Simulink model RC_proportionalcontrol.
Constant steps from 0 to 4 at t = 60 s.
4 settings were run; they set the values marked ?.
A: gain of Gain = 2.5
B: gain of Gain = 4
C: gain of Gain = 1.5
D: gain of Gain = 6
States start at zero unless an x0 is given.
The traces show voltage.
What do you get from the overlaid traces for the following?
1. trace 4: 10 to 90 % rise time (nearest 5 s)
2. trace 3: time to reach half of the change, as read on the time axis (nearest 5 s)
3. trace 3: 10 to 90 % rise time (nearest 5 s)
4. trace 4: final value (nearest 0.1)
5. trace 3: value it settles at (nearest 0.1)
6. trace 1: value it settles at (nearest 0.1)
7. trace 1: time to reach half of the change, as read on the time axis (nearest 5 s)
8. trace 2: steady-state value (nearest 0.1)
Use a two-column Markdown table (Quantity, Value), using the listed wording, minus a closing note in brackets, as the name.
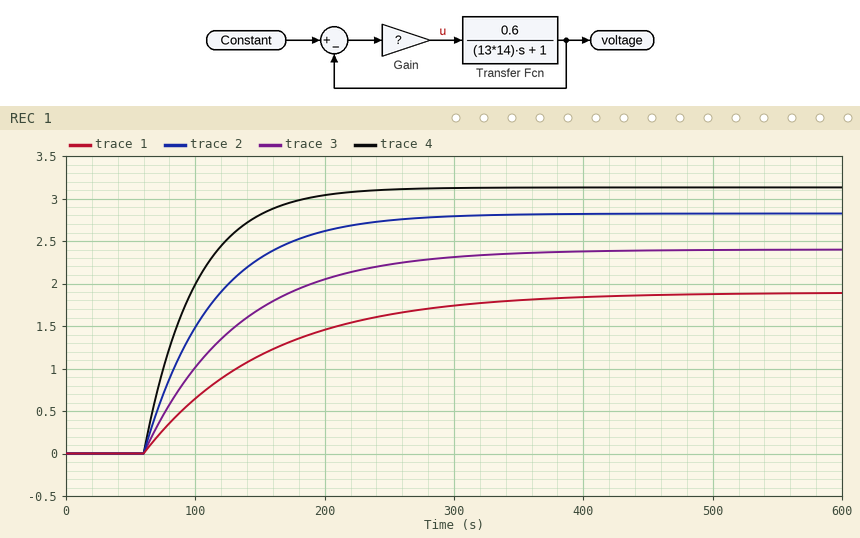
| Quantity | Value |
|---|---|
| trace 4: 10 to 90 % rise time | 85 s |
| trace 3: time to reach half of the change, as read on the time axis | 110 s |
| trace 3: 10 to 90 % rise time | 160 s |
| trace 4: final value | 3.1 |
| trace 3: value it settles at | 2.4 |
| trace 1: value it settles at | 1.9 |
| trace 1: time to reach half of the change, as read on the time axis | 125 s |
| trace 2: steady-state value | 2.8 |
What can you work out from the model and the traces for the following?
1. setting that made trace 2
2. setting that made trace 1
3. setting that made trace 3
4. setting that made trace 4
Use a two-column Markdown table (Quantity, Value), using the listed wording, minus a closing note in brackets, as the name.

| Quantity | Value |
|---|---|
| setting that made trace 2 | B |
| setting that made trace 1 | C |
| setting that made trace 3 | A |
| setting that made trace 4 | D |
